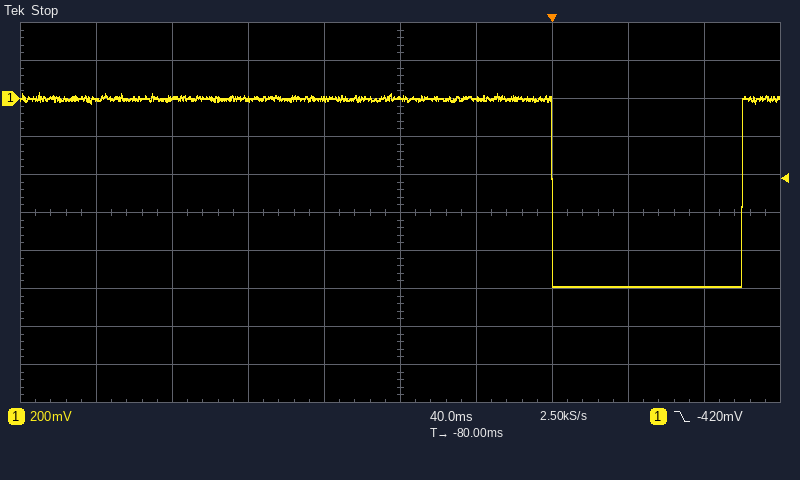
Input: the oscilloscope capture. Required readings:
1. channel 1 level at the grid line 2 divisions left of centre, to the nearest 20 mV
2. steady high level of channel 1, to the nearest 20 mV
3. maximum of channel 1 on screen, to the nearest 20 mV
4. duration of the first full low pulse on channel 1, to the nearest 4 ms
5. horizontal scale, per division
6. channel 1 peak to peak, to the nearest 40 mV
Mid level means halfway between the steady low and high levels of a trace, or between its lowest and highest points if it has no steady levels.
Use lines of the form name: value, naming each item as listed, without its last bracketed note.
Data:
channel 1 level at the grid line 2 divisions left of centre, to the nearest 20 mV: 0 mV
steady high level of channel 1, to the nearest 20 mV: 0 mV
maximum of channel 1 on screen, to the nearest 20 mV: 40 mV
duration of the first full low pulse on channel 1, to the nearest 4 ms: 100 ms
horizontal scale, per division: 40 ms
channel 1 peak to peak, to the nearest 40 mV: 1.04 V
